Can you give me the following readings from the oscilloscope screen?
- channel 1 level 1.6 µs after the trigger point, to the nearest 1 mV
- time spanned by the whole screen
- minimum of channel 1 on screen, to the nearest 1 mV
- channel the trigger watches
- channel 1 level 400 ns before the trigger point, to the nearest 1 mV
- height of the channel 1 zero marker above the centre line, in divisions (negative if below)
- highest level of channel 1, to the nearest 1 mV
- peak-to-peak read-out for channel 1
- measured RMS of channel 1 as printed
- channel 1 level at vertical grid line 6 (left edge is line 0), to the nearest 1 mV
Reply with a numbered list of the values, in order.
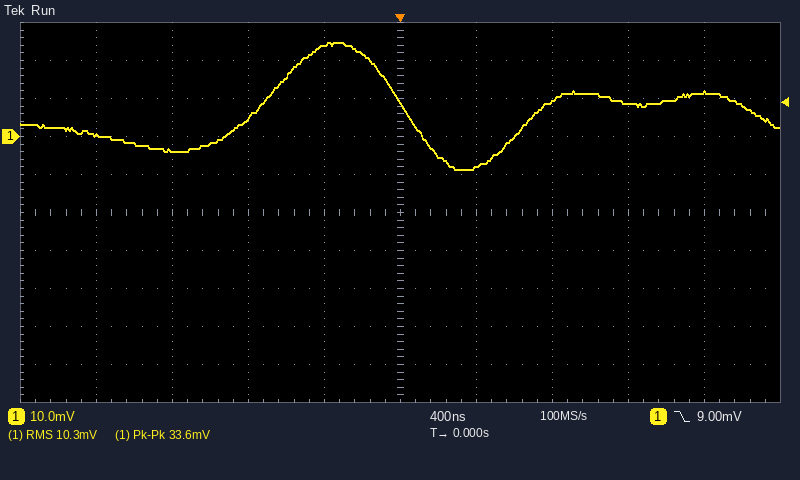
1. 12 mV
2. 4 µs
3. -9 mV
4. channel 1
5. 24 mV
6. +2.0 div
7. 25 mV
8. 33.6 mV
9. 10.3 mV
10. -8 mV
